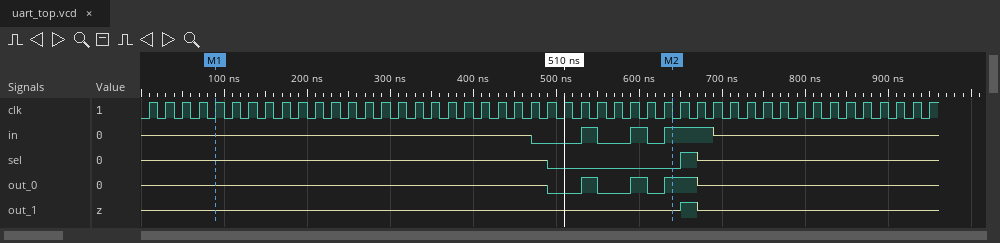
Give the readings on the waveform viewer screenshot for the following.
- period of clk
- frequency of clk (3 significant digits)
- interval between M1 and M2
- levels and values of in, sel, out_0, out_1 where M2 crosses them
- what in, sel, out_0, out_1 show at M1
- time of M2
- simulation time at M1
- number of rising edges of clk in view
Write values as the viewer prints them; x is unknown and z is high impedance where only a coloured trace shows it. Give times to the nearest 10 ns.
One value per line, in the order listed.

20 ns
50.0 MHz
550 ns
in=1, sel=0, out_0=1, out_1=z
in=z, sel=z, out_0=z, out_1=z
640 ns
90 ns
48
